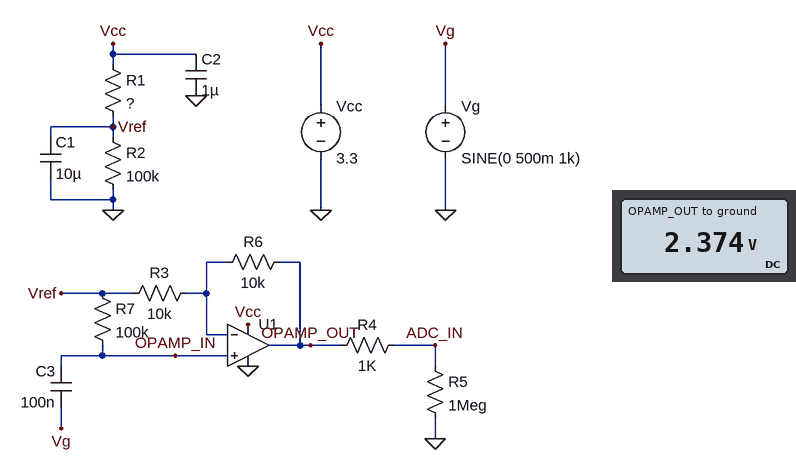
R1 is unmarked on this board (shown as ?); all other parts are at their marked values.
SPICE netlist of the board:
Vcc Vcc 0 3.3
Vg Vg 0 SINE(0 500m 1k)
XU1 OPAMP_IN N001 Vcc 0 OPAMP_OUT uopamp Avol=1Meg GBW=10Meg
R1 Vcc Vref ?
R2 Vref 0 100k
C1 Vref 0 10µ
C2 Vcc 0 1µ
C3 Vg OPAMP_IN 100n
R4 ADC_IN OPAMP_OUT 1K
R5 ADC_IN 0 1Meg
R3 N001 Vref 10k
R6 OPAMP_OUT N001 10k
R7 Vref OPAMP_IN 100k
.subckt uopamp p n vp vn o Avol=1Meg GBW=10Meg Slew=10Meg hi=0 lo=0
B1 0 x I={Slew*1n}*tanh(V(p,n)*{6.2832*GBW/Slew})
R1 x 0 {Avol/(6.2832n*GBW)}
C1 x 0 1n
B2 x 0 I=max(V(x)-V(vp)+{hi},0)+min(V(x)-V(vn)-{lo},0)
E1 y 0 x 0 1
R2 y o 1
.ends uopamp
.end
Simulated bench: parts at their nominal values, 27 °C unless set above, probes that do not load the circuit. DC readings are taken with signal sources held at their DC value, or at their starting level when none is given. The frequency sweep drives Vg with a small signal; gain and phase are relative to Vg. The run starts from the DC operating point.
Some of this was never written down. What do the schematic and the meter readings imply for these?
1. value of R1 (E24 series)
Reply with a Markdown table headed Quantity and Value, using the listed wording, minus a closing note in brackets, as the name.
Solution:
| Quantity | Value |
|---|---|
| value of R1 | 39 kΩ |
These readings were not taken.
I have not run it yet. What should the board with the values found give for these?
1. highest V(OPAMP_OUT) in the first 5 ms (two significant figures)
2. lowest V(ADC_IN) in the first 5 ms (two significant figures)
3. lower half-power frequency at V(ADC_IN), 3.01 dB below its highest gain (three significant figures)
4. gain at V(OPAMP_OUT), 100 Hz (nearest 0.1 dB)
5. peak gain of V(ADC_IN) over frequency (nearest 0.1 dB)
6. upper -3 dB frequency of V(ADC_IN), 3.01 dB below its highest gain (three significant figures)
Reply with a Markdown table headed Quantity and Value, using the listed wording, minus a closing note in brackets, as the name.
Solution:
| Quantity | Value |
|---|---|
| highest V(OPAMP_OUT) in the first 5 ms | 3.3 V |
| lowest V(ADC_IN) in the first 5 ms | 1.4 V |
| lower half-power frequency at V(ADC_IN), 3.01 dB below its highest gain | 17.6 Hz |
| gain at V(OPAMP_OUT), 100 Hz | 5.9 dB |
| peak gain of V(ADC_IN) over frequency | 6.0 dB |
| upper -3 dB frequency of V(ADC_IN), 3.01 dB below its highest gain | 5.00 MHz |
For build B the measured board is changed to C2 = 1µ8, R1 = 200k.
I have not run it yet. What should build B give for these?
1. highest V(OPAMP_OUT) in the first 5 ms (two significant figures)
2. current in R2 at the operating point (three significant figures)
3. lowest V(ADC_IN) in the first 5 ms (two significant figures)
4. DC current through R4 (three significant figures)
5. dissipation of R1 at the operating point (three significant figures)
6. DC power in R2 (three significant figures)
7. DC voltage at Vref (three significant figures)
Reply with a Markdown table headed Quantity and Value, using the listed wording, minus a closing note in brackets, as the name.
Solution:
| Quantity | Value |
|---|---|
| highest V(OPAMP_OUT) in the first 5 ms | 2.1 V |
| current in R2 at the operating point | 11.0 µA |
| lowest V(ADC_IN) in the first 5 ms | 85 mV |
| DC current through R4 | 1.10 µA |
| dissipation of R1 at the operating point | 24.2 µW |
| DC power in R2 | 12.1 µW |
| DC voltage at Vref | 1.10 V |
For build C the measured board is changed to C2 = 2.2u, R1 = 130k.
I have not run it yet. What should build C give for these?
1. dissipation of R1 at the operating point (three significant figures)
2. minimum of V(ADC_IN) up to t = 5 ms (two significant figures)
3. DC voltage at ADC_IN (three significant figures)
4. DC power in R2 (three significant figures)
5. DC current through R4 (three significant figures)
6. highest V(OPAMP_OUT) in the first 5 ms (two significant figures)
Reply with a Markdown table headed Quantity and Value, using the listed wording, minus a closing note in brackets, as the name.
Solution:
| Quantity | Value |
|---|---|
| dissipation of R1 at the operating point | 26.8 µW |
| minimum of V(ADC_IN) up to t = 5 ms | 420 mV |
| DC voltage at ADC_IN | 1.43 V |
| DC power in R2 | 20.6 µW |
| DC current through R4 | 1.43 µA |
| highest V(OPAMP_OUT) in the first 5 ms | 2.4 V |
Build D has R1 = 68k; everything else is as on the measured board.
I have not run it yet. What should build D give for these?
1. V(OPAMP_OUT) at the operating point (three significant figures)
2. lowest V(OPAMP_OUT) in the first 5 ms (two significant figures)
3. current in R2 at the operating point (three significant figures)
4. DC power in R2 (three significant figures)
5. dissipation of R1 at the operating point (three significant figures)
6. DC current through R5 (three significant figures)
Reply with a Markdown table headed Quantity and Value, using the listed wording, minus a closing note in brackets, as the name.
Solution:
| Quantity | Value |
|---|---|
| V(OPAMP_OUT) at the operating point | 1.96 V |
| lowest V(OPAMP_OUT) in the first 5 ms | 950 mV |
| current in R2 at the operating point | 19.6 µA |
| DC power in R2 | 38.6 µW |
| dissipation of R1 at the operating point | 26.2 µW |
| DC current through R5 | 1.96 µA |
